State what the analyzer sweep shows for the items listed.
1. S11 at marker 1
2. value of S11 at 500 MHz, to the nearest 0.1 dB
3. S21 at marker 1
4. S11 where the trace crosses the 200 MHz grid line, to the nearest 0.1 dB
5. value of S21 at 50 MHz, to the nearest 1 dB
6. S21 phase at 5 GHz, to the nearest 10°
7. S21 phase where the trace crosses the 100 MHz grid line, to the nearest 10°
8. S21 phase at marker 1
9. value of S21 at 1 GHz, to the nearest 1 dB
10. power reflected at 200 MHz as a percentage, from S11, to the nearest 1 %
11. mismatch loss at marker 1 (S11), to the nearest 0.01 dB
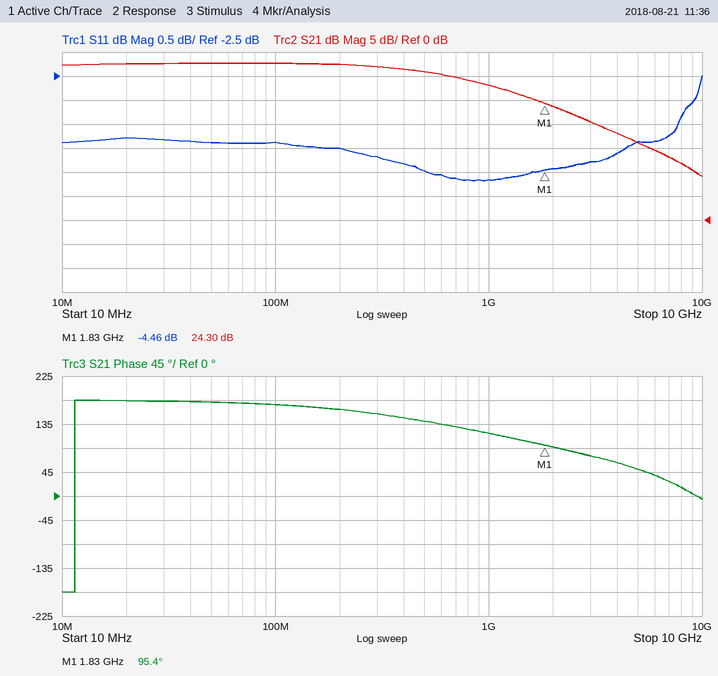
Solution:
-4.46 dB
-4.5 dB
24.30 dB
-4.0 dB
33 dB
50°
170°
95.4°
28 dB
40 %
1.93 dB
